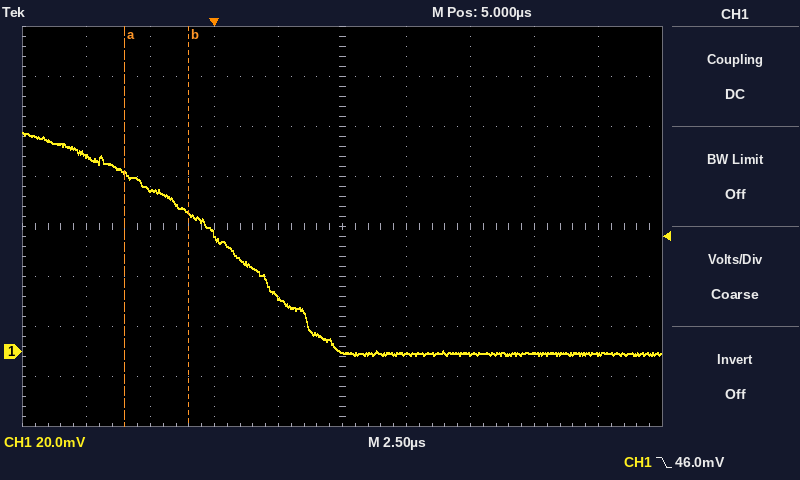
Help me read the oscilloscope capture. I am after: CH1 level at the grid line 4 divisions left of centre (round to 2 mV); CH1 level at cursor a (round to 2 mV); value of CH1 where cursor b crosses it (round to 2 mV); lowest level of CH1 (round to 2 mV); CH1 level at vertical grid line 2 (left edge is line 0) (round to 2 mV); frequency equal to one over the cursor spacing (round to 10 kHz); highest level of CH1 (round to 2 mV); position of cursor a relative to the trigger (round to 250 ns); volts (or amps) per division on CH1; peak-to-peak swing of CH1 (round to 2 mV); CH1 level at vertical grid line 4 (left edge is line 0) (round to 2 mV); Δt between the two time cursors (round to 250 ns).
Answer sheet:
78 mV
72 mV
56 mV
-2 mV
64 mV
400 kHz
88 mV
-3.50 µs
20 mV
90 mV
22 mV
2.50 µs
